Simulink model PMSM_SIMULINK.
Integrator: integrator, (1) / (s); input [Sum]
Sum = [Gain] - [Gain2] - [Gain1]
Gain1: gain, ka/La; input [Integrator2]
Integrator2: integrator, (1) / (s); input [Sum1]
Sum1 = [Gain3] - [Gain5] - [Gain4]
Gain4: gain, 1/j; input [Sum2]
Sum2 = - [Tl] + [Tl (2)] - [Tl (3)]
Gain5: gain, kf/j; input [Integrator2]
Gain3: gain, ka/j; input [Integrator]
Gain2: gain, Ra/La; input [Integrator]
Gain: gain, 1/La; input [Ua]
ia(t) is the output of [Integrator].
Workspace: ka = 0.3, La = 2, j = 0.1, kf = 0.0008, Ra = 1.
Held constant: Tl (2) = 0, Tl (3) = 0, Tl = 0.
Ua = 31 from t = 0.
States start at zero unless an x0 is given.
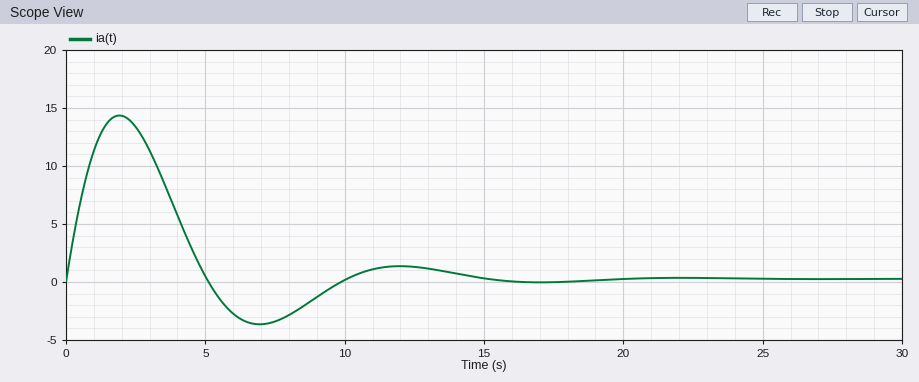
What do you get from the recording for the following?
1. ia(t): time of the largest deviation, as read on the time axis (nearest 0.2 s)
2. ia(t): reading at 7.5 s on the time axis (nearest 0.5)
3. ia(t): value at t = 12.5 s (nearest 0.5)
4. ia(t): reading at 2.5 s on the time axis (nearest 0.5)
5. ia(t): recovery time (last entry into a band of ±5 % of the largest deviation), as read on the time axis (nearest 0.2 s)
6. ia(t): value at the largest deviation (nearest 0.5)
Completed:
2.0 s
-3.5
1.5
13.5
13.4 s
14.5
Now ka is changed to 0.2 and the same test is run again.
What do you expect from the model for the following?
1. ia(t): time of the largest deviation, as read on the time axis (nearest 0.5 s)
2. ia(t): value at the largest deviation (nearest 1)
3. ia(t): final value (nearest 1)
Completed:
2.5 s
18
1
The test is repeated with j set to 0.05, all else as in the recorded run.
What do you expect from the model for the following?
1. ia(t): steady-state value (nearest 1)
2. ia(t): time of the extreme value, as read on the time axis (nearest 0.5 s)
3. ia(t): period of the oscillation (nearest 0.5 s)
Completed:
0
1.5 s
7.0 s
